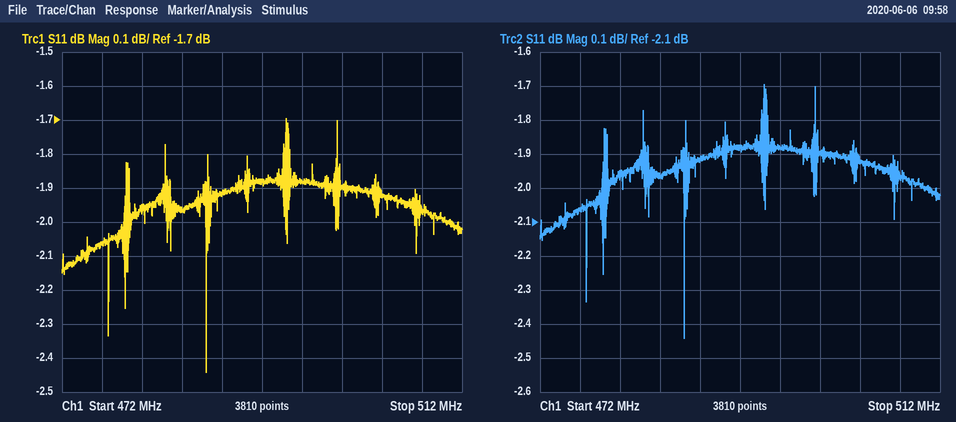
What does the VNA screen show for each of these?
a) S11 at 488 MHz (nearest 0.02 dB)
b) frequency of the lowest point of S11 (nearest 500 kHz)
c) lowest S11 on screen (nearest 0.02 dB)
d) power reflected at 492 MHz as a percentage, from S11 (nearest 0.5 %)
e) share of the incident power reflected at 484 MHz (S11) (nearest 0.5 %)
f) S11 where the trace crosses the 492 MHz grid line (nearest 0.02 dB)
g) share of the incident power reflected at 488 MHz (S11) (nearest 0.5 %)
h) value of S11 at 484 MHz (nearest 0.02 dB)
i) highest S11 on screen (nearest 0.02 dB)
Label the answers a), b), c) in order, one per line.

a) -1.92 dB
b) 486.5 MHz
c) -2.44 dB
d) 65.0 %
e) 63.5 %
f) -1.88 dB
g) 64.5 %
h) -1.96 dB
i) -1.70 dB
